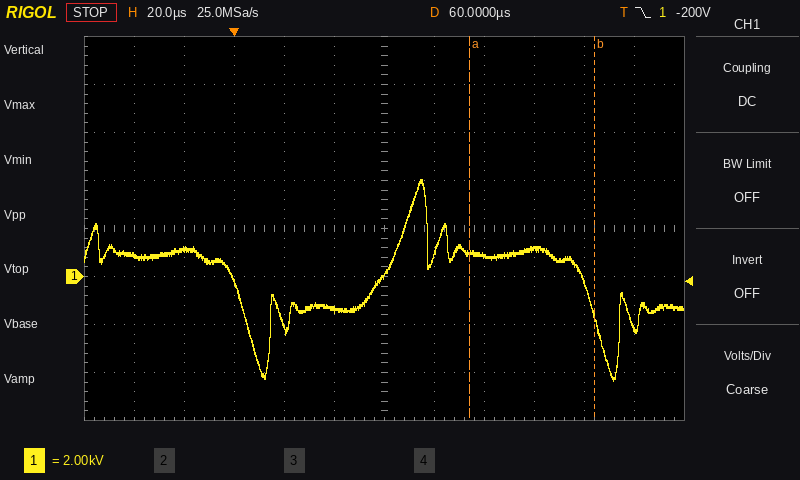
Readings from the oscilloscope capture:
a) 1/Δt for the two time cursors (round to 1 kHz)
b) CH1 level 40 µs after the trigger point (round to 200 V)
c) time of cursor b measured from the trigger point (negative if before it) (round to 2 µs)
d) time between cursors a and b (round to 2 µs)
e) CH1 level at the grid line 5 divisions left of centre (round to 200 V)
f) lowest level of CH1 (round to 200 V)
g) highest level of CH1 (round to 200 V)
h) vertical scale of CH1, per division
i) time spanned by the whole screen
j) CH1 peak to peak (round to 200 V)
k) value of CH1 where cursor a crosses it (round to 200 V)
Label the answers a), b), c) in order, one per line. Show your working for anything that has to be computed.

a) 1 / 50 µs ≈ 20 kHz
b) -1.4 kV
c) +144 µs
d) 50 µs
e) 800 V
f) -4.4 kV
g) 4.0 kV
h) 2 kV
i) 240 µs
j) 4.0 kV − (-4.4 kV) = 8.4 kV
k) 1.0 kV
